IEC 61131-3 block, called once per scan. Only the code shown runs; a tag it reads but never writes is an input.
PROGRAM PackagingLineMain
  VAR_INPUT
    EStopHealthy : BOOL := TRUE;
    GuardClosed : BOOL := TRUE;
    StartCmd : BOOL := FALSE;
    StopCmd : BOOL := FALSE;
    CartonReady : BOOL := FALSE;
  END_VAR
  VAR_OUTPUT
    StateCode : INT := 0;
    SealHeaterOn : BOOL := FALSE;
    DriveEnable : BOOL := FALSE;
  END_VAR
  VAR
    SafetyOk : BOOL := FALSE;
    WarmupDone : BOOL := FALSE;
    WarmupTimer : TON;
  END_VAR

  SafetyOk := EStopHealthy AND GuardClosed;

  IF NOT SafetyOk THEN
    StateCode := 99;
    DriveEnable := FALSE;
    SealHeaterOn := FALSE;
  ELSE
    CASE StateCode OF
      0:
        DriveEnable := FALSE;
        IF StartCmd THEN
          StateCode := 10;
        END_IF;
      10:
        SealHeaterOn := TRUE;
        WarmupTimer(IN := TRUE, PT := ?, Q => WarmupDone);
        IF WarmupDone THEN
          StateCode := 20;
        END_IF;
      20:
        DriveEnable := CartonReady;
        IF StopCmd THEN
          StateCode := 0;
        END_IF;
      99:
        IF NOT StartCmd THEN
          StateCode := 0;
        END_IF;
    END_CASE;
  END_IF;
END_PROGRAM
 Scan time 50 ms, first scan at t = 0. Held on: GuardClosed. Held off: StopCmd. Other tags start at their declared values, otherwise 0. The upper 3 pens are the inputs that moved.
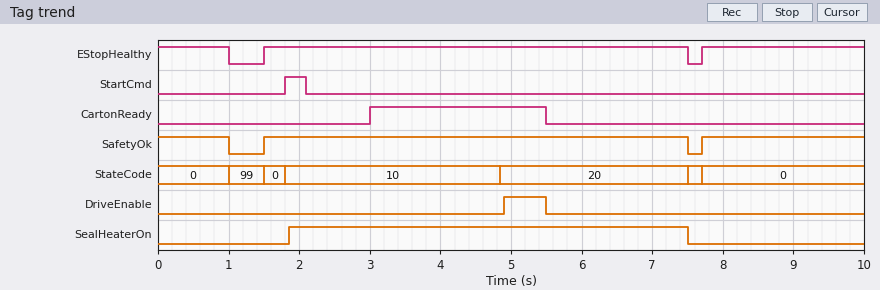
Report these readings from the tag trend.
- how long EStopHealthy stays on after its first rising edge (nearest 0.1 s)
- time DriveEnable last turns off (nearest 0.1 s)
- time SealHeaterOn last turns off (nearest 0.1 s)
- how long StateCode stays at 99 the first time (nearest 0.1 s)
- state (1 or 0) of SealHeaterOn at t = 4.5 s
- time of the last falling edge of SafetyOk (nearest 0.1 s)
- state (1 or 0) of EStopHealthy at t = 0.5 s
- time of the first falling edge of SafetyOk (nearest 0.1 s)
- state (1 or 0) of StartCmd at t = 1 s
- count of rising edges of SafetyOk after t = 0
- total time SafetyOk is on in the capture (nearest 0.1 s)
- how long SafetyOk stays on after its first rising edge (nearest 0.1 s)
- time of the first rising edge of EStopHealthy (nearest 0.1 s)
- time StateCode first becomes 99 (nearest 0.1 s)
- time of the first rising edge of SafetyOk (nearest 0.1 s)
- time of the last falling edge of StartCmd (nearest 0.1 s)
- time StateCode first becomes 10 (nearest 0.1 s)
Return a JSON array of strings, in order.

["6.0 s", "5.5 s", "7.5 s", "0.5 s", "1", "7.5 s", "1", "1.0 s", "0", "2", "9.3 s", "6.0 s", "1.5 s", "1.0 s", "1.5 s", "2.1 s", "1.8 s"]
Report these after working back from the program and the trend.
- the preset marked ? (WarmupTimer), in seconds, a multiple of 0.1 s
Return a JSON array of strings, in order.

["3.0 s"]
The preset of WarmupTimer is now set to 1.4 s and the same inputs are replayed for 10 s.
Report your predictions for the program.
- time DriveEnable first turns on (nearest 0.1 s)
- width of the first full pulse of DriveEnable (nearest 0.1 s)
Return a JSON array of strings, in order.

["3.3 s", "2.2 s"]
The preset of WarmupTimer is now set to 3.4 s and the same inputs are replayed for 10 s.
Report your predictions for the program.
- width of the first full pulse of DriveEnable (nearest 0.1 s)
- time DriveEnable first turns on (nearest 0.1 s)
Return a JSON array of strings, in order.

["0.2 s", "5.3 s"]
